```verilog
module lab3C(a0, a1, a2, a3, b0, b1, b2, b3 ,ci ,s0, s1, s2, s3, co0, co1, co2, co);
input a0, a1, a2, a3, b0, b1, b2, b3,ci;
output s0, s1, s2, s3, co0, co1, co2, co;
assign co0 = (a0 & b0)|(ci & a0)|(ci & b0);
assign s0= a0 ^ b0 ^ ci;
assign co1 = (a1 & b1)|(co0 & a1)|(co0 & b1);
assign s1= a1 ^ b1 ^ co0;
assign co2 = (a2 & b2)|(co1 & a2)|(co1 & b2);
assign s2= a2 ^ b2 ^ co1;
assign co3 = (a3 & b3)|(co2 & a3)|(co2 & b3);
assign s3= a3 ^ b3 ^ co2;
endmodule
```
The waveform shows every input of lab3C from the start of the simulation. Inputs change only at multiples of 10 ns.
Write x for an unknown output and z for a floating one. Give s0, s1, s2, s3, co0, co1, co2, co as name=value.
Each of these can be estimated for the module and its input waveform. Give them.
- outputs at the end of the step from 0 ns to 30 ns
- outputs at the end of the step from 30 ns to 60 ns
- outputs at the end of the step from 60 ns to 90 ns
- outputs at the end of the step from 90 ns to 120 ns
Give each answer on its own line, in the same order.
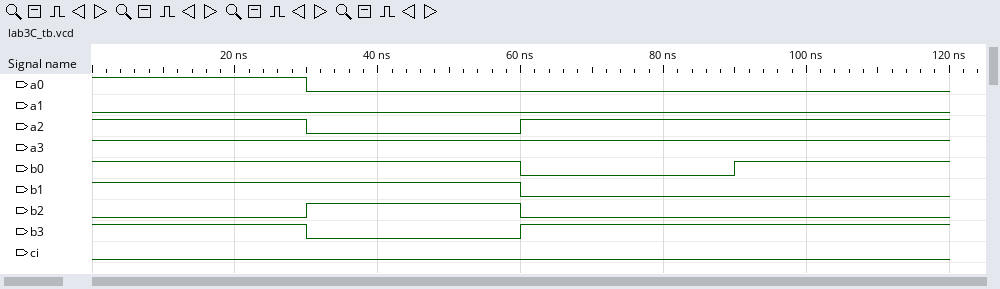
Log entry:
s0=0, s1=0, s2=0, s3=1, co0=1, co1=1, co2=1, co=z
s0=1, s1=1, s2=1, s3=1, co0=0, co1=0, co2=0, co=z
s0=0, s1=0, s2=1, s3=0, co0=0, co1=0, co2=0, co=z
s0=1, s1=0, s2=1, s3=0, co0=0, co1=0, co2=0, co=z
